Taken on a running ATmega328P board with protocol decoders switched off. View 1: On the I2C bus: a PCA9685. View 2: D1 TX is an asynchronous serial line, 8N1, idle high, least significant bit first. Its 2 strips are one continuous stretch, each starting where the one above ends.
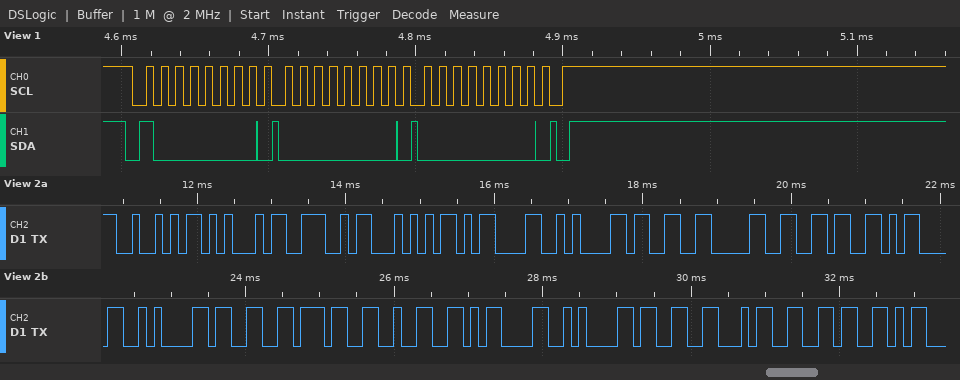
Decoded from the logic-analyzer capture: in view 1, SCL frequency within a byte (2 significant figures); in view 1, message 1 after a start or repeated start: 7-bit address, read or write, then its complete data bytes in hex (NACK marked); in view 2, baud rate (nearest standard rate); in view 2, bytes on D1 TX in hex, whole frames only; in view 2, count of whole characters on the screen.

100 kHz
0x40 write: 00 00
9600 baud
0x52 0x45 0x4E 0x54 0x0D 0x0A 0x33 0x30 0x36 0x0D 0x0A 0x33 0x37 0x32 0x0D 0x0A 0x33 0x34 0x36
19
